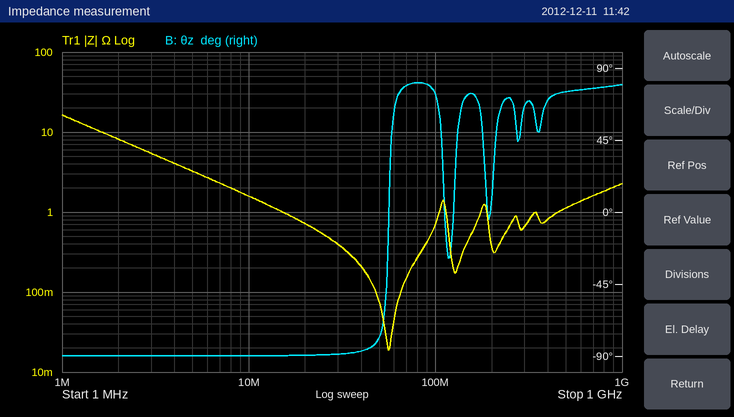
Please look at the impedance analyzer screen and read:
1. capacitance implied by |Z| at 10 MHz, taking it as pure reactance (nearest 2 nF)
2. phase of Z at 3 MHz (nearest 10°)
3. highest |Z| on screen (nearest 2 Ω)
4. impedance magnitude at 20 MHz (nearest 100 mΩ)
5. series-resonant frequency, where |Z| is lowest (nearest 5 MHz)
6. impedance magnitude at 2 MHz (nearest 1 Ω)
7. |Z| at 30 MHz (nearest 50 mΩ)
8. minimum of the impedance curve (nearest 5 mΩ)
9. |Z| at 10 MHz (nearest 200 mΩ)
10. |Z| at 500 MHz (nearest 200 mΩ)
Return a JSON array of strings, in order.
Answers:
["10 nF", "-90°", "16 Ω", "700 mΩ", "55 MHz", "8 Ω", "400 mΩ", "20 mΩ", "1.6 Ω", "1.2 Ω"]
